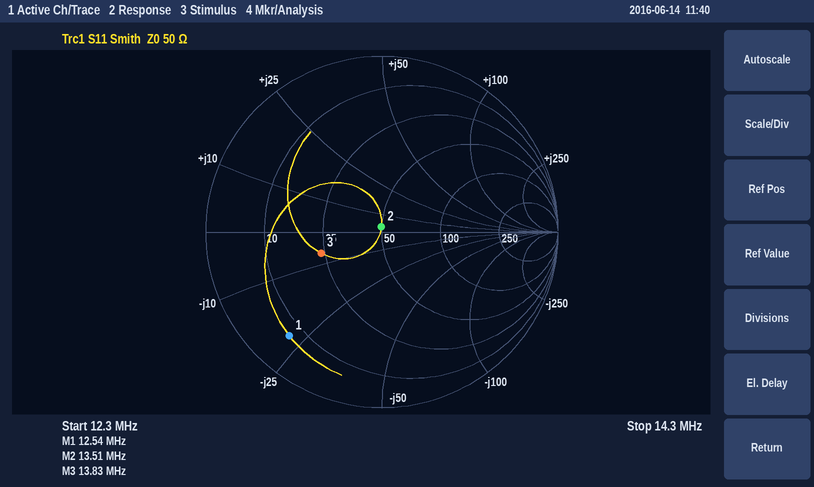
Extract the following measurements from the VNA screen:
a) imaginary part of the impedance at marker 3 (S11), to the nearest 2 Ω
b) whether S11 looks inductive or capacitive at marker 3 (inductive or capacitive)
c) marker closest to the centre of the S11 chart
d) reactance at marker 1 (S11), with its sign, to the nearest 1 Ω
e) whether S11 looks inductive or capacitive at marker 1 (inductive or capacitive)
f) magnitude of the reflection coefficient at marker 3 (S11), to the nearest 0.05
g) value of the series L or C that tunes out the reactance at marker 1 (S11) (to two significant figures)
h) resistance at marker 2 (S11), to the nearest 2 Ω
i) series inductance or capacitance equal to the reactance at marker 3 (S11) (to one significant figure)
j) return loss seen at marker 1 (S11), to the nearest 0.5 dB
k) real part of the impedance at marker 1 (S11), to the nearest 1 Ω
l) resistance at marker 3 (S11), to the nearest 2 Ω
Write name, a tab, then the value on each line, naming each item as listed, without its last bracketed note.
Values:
imaginary part of the impedance at marker 3 (S11), to the nearest 2 Ω	-6 Ω
whether S11 looks inductive or capacitive at marker 3	capacitive
marker closest to the centre of the S11 chart	marker 2
reactance at marker 1 (S11), with its sign, to the nearest 1 Ω	-22 Ω
whether S11 looks inductive or capacitive at marker 1	capacitive
magnitude of the reflection coefficient at marker 3 (S11), to the nearest 0.05	0.35
value of the series L or C that tunes out the reactance at marker 1 (S11)	280 nH
resistance at marker 2 (S11), to the nearest 2 Ω	50 Ω
series inductance or capacitance equal to the reactance at marker 3 (S11)	2 nF
return loss seen at marker 1 (S11), to the nearest 0.5 dB	2.0 dB
real part of the impedance at marker 1 (S11), to the nearest 1 Ω	7 Ω
resistance at marker 3 (S11), to the nearest 2 Ω	24 Ω
